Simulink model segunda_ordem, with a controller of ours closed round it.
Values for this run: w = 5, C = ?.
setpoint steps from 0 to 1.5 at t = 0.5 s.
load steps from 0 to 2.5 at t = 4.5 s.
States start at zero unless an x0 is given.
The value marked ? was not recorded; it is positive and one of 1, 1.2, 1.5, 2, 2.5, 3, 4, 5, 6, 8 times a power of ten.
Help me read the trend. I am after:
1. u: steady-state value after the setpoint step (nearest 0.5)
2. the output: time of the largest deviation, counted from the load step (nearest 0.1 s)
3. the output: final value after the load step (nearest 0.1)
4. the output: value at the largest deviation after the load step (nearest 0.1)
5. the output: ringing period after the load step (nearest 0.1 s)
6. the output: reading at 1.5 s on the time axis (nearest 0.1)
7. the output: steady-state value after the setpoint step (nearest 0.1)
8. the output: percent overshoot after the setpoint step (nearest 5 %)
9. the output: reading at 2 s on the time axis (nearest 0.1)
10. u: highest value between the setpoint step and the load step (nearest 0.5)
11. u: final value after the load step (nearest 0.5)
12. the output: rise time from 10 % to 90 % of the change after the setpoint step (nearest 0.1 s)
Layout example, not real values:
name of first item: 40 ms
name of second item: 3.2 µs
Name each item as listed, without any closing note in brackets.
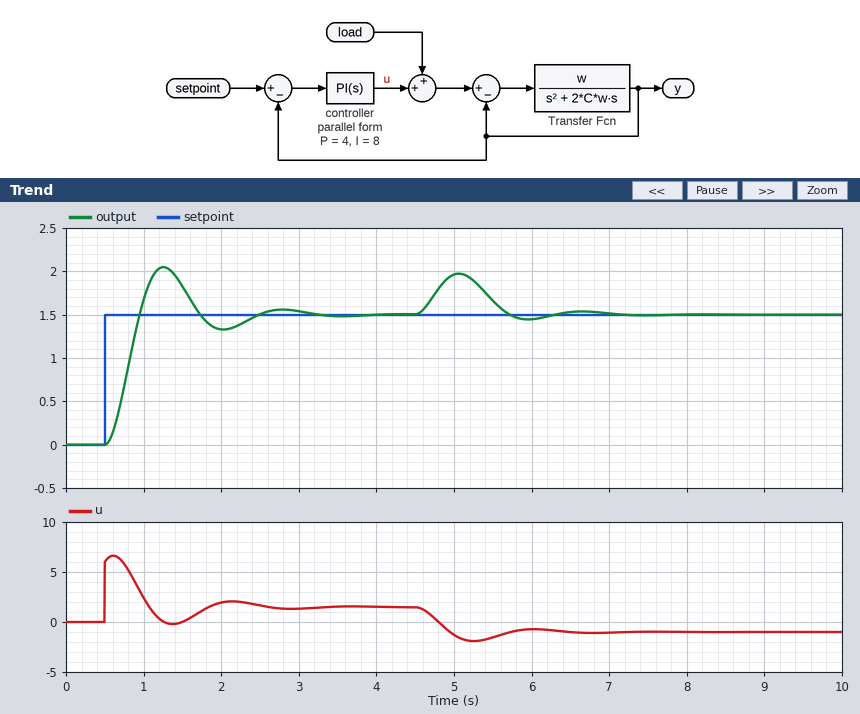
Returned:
u: steady-state value after the setpoint step: 1.5
the output: time of the largest deviation, counted from the load step: 0.6 s
the output: final value after the load step: 1.5
the output: value at the largest deviation after the load step: 2.0
the output: ringing period after the load step: 1.6 s
the output: reading at 1.5 s on the time axis: 1.8
the output: steady-state value after the setpoint step: 1.5
the output: percent overshoot after the setpoint step: 35 %
the output: reading at 2 s on the time axis: 1.3
u: highest value between the setpoint step and the load step: 6.5
u: final value after the load step: -1.0
the output: rise time from 10 % to 90 % of the change after the setpoint step: 0.3 s
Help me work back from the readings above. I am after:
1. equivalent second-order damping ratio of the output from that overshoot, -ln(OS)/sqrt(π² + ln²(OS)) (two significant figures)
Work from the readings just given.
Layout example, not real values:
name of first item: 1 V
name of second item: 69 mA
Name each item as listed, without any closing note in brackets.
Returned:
equivalent second-order damping ratio of the output from that overshoot, -ln(OS)/sqrt(π² + ln²(OS)): 0.32
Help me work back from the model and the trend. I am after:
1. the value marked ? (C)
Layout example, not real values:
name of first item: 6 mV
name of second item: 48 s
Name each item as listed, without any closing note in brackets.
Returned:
the value marked ?: 0.5
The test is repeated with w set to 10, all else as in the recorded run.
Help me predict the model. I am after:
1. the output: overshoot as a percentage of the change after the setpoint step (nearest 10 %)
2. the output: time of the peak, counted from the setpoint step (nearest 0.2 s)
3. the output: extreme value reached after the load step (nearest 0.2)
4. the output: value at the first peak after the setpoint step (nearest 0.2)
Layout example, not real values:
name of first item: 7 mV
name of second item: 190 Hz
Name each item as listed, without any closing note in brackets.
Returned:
the output: overshoot as a percentage of the change after the setpoint step: 20 %
the output: time of the peak, counted from the setpoint step: 0.6 s
the output: extreme value reached after the load step: 2.0
the output: value at the first peak after the setpoint step: 1.8
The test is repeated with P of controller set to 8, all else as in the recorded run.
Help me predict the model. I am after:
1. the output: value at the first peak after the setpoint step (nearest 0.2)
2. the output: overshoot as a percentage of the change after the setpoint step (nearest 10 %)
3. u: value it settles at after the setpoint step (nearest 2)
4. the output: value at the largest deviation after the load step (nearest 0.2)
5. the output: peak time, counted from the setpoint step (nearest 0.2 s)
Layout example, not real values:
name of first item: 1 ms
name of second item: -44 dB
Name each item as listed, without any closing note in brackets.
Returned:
the output: value at the first peak after the setpoint step: 2.0
the output: overshoot as a percentage of the change after the setpoint step: 30 %
u: value it settles at after the setpoint step: 2
the output: value at the largest deviation after the load step: 1.8
the output: peak time, counted from the setpoint step: 0.6 s
